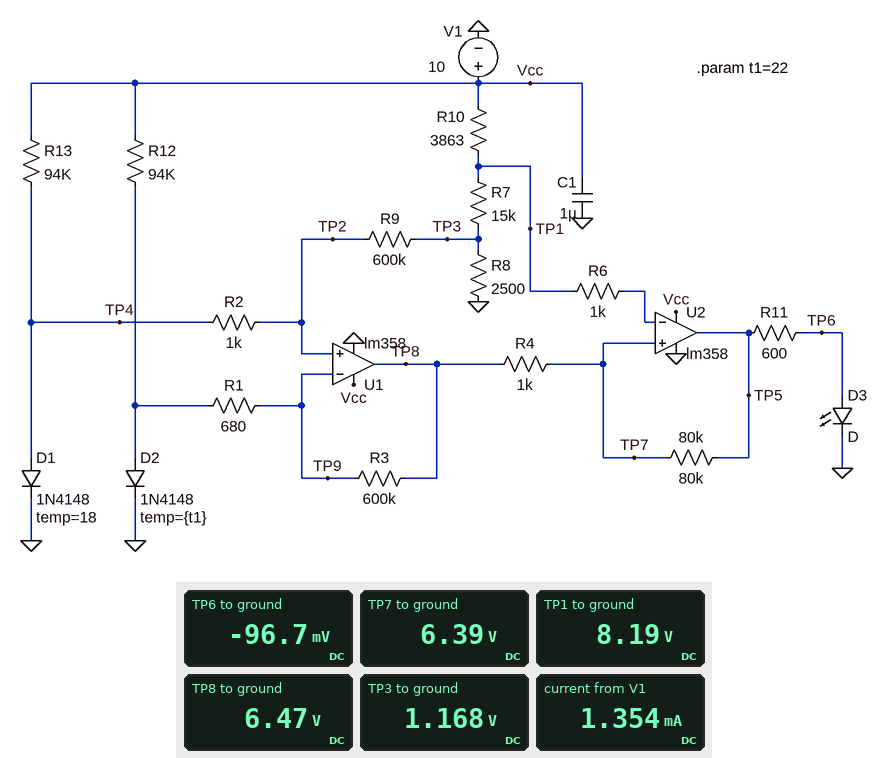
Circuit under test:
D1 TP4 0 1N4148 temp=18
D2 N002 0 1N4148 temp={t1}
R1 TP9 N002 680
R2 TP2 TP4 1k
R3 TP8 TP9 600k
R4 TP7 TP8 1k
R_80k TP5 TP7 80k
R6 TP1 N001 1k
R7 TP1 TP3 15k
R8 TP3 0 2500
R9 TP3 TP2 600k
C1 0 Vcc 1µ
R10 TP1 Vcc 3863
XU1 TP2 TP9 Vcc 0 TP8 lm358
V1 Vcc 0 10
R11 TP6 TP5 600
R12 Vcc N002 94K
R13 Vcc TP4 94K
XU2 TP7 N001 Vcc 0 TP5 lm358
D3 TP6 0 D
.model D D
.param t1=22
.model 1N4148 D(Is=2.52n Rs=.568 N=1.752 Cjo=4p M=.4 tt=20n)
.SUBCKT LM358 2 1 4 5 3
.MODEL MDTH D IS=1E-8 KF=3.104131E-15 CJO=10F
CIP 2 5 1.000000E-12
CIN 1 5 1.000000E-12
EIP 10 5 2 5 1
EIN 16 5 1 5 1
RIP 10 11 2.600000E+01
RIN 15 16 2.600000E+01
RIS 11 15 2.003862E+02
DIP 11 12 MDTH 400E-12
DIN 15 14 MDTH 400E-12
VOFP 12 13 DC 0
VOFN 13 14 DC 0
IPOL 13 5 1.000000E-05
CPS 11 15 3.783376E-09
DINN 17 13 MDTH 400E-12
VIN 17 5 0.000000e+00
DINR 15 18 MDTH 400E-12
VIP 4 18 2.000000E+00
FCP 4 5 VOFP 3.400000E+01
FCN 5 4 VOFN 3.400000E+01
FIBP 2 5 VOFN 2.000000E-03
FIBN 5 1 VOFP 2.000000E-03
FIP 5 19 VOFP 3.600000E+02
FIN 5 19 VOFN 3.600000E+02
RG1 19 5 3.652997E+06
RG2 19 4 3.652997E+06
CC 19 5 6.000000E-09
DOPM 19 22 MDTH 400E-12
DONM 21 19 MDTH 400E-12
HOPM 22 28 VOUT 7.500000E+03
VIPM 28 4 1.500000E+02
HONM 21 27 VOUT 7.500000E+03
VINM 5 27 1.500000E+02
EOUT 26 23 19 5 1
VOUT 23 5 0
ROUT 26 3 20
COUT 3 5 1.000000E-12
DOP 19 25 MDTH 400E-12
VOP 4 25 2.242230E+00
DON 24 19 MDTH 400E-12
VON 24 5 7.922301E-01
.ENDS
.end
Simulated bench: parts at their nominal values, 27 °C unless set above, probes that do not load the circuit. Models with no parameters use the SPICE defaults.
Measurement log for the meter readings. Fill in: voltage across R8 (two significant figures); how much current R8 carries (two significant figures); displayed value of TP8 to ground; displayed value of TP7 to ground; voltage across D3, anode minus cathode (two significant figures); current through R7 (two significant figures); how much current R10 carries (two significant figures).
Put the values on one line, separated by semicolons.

1.2 V; 470 µA; 6.47 V; 6.39 V; -97 mV; 470 µA; 470 µA
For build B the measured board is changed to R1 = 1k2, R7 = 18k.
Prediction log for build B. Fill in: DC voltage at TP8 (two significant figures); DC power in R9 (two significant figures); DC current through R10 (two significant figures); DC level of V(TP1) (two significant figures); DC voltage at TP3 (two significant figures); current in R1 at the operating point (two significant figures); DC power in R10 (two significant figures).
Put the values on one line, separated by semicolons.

4.4 V; 450 nW; 410 µA; 8.4 V; 1.0 V; 6.5 µA; 650 µW
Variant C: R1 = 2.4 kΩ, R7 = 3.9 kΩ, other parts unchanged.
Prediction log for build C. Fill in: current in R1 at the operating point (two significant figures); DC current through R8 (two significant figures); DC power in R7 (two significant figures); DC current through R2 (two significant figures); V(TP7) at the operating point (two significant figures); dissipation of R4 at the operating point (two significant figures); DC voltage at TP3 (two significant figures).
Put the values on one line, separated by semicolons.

4.9 µA; 970 µA; 3.7 mW; 3.2 µA; 3.4 V; 1.9 µW; 2.4 V
